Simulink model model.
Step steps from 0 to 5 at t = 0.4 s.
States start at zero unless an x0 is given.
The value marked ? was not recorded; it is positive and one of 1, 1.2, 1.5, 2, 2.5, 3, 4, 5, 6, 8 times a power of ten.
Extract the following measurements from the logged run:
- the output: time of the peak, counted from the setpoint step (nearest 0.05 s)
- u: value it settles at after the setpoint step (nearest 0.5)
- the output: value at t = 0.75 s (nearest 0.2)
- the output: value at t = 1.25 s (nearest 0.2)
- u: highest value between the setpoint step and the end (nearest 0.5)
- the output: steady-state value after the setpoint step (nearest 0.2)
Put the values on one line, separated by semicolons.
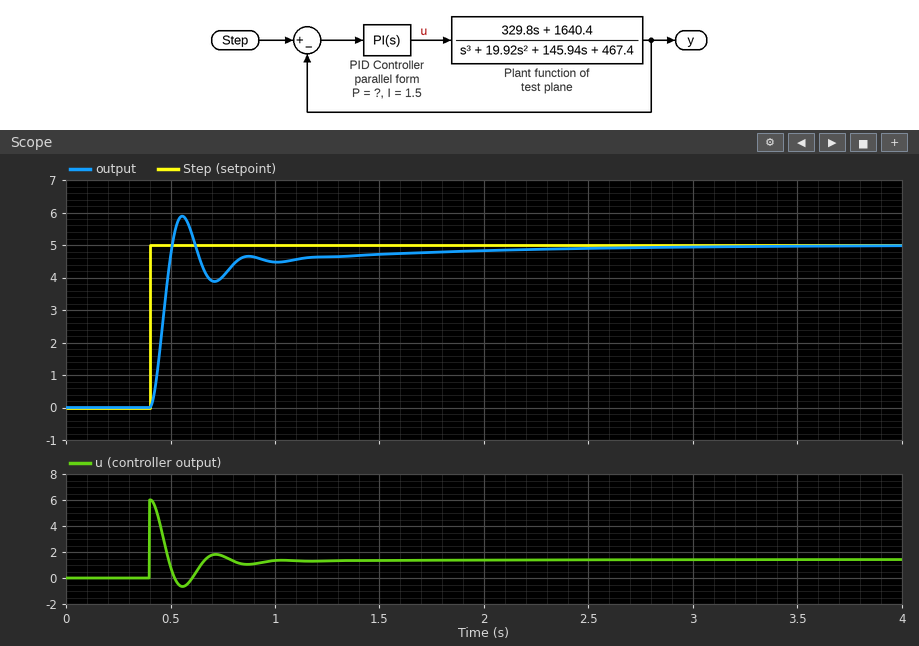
0.15 s; 1.5; 4.0; 4.6; 6.0; 5.0
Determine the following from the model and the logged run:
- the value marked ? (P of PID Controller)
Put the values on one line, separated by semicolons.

1.2
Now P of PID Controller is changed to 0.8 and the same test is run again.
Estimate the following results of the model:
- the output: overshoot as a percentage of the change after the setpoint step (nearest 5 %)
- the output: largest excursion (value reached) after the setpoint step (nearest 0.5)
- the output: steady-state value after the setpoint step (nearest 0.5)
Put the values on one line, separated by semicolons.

10 %; 5.5; 5.0
